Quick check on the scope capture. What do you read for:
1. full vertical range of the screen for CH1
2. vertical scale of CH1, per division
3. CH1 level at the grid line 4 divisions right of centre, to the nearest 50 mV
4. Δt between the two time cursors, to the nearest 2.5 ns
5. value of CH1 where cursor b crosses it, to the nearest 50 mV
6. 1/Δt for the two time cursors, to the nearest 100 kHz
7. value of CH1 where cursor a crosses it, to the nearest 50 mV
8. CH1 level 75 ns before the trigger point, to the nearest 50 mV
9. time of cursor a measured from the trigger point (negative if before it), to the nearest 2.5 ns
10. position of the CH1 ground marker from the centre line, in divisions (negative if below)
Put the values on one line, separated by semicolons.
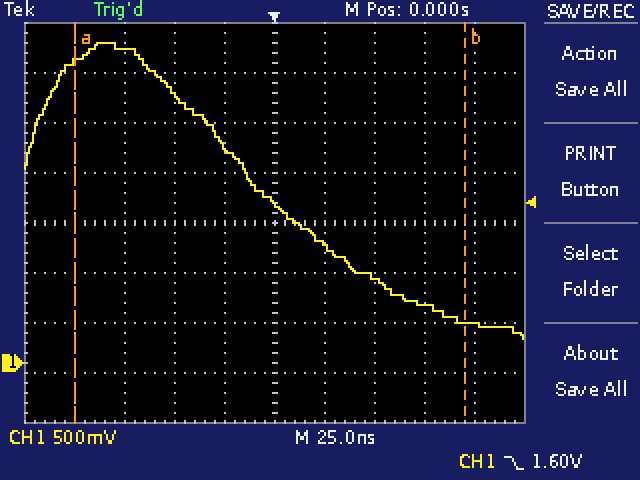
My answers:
4 V; 500 mV; 400 mV; 195.0 ns; 400 mV; 5.1 MHz; 3.00 V; 3.15 V; -100.0 ns; -2.8 div
